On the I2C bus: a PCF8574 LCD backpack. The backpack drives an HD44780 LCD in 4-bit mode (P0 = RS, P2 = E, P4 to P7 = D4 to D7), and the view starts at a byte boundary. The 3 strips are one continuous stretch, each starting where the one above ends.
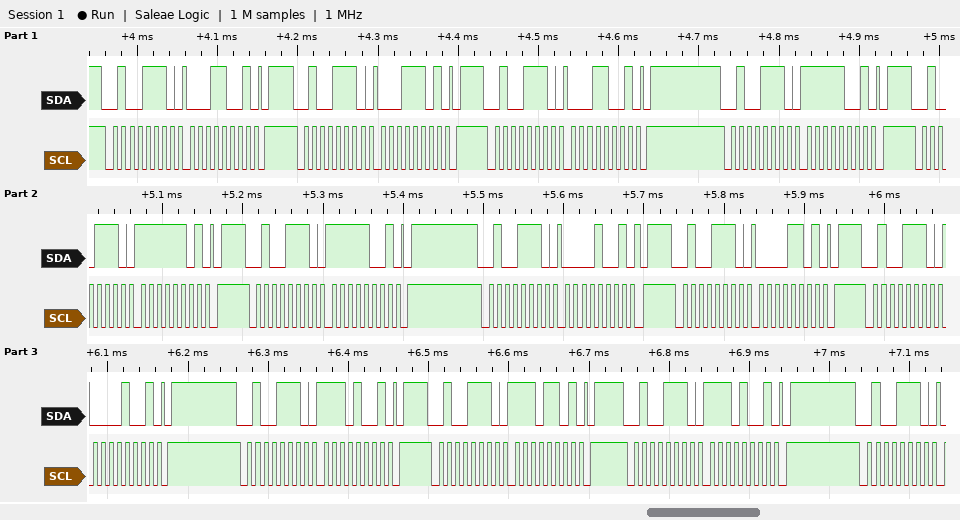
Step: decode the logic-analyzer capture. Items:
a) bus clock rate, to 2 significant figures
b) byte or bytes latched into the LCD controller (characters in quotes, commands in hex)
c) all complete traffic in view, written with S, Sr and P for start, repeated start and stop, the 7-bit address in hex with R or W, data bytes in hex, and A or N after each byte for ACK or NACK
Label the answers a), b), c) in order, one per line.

a) 100 kHz
b) data 0x1F data 0x0E
c) S 27W A 19 A P S 27W A 1D A P S 27W A 19 A P S 27W A F9 A P S 27W A FD A P S 27W A F9 A P S 27W A 09 A P S 27W A 0D A P S 27W A 09 A P S 27W A E9 A P S 27W A ED A P S 27W A E9 A P S 27W A
